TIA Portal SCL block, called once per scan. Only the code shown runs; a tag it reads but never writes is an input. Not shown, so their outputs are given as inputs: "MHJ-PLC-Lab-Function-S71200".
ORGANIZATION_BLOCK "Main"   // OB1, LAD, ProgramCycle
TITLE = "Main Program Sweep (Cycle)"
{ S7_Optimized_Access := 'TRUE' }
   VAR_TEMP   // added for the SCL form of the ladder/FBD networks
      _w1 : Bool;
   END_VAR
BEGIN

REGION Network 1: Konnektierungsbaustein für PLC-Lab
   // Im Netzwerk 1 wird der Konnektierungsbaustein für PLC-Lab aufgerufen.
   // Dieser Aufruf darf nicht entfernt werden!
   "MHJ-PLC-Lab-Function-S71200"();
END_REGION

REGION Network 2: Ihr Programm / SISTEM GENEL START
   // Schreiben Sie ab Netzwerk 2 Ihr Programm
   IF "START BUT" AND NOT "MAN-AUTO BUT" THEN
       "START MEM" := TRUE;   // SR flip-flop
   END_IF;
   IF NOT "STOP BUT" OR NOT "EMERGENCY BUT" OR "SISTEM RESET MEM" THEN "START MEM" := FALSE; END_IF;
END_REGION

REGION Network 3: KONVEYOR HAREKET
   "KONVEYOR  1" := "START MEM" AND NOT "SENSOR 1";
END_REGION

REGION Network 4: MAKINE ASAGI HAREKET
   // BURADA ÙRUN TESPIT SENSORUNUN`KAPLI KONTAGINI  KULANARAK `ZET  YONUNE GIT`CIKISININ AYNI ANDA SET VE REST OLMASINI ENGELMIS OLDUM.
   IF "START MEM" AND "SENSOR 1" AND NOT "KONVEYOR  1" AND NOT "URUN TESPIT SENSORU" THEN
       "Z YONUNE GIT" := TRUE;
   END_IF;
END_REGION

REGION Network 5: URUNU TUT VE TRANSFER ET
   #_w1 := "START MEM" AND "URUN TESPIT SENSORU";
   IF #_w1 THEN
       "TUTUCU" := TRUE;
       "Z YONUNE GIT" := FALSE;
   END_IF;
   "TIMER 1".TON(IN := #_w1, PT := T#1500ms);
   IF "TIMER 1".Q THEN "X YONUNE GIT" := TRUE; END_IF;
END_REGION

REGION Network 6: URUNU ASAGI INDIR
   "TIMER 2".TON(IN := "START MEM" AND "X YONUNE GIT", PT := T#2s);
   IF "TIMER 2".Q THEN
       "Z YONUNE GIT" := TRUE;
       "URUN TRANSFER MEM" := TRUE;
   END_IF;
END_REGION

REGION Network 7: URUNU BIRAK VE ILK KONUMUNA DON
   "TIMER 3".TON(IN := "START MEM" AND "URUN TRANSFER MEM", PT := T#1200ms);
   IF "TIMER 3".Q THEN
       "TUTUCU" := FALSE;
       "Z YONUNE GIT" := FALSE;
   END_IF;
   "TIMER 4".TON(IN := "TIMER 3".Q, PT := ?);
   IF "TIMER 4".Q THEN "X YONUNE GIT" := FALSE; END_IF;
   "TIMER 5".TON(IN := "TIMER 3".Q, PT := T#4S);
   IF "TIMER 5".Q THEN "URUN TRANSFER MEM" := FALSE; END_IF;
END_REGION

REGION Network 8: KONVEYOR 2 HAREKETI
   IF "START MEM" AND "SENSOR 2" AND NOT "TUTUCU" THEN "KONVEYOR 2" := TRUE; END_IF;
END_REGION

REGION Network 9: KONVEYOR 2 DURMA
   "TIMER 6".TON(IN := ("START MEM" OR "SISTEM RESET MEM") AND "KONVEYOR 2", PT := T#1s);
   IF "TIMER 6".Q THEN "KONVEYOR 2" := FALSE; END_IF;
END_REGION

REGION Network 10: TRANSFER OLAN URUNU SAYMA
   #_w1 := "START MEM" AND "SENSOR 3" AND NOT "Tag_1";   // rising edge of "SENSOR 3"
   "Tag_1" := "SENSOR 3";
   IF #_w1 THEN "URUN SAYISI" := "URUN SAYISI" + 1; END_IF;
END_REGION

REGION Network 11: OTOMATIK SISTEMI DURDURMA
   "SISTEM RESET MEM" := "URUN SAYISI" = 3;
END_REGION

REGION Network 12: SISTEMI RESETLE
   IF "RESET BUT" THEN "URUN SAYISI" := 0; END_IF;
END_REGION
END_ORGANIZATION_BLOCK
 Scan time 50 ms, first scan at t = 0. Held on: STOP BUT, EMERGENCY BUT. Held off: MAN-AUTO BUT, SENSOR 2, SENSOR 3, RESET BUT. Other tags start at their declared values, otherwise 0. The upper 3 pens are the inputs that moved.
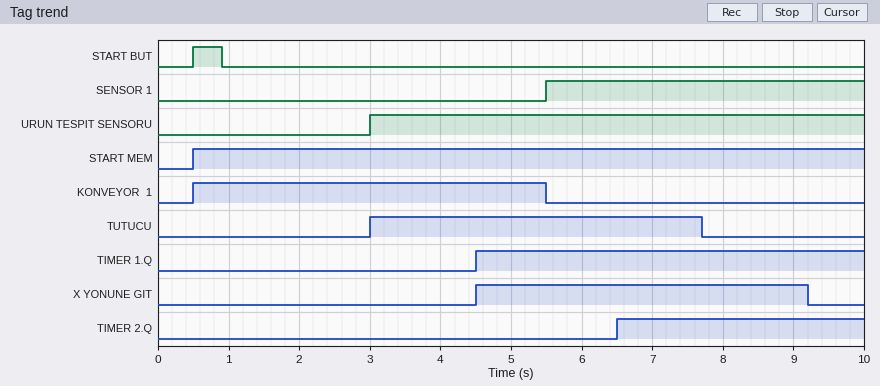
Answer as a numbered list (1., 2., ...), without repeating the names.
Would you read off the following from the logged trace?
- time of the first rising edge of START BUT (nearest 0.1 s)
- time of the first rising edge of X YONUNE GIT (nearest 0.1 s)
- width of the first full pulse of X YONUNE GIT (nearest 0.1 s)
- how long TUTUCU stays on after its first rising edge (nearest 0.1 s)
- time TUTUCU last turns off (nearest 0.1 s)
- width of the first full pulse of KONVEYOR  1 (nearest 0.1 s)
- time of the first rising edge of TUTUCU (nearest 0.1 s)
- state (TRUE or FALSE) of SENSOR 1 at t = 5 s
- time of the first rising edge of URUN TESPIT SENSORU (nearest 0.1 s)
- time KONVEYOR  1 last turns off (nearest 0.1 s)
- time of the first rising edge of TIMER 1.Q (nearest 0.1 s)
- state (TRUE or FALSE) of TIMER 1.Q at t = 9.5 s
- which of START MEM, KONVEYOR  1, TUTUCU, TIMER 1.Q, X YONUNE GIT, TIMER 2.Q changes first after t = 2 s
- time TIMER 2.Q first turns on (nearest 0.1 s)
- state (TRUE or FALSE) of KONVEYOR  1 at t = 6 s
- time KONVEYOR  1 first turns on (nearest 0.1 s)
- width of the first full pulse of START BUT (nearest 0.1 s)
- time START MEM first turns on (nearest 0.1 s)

1. 0.5 s
2. 4.5 s
3. 4.7 s
4. 4.7 s
5. 7.7 s
6. 5.0 s
7. 3.0 s
8. FALSE
9. 3.0 s
10. 5.5 s
11. 4.5 s
12. TRUE
13. TUTUCU
14. 6.5 s
15. FALSE
16. 0.5 s
17. 0.4 s
18. 0.5 s
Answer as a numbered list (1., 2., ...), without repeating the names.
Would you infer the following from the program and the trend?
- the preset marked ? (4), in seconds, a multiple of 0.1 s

1. 1.5 s
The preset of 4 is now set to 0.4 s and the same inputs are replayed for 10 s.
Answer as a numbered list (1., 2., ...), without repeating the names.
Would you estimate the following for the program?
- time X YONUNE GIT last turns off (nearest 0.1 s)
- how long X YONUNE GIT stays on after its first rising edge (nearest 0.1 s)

1. 8.1 s
2. 3.6 s
